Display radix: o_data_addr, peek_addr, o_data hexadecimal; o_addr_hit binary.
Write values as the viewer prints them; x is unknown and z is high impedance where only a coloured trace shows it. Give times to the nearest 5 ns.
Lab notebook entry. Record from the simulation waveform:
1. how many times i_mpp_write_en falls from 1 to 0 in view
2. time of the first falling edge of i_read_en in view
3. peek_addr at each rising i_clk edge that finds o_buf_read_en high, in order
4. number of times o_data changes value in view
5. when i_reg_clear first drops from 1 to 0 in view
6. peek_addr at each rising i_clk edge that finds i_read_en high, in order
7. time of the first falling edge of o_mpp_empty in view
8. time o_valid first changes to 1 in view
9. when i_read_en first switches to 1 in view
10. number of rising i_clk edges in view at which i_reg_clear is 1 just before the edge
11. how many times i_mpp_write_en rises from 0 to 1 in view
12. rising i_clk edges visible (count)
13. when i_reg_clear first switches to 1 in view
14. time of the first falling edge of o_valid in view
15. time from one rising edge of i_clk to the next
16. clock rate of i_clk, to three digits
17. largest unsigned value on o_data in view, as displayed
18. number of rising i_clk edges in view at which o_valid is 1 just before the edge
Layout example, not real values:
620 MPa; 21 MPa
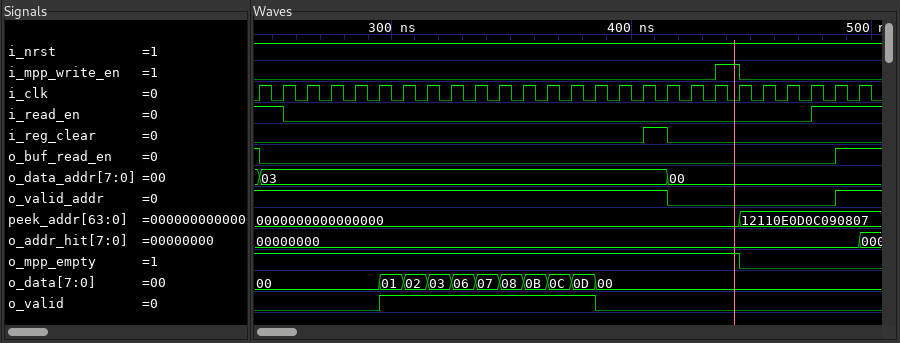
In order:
1; 255 ns; 0000000000000000, 12110E0D0C090807; 10; 415 ns; 0000000000000000, 0000000000000000, 12110E0D0C090807, 12110E0D0C090807; 445 ns; 295 ns; 475 ns; 1; 1; 26; 405 ns; 385 ns; 10 ns; 100 MHz; 0D; 9
